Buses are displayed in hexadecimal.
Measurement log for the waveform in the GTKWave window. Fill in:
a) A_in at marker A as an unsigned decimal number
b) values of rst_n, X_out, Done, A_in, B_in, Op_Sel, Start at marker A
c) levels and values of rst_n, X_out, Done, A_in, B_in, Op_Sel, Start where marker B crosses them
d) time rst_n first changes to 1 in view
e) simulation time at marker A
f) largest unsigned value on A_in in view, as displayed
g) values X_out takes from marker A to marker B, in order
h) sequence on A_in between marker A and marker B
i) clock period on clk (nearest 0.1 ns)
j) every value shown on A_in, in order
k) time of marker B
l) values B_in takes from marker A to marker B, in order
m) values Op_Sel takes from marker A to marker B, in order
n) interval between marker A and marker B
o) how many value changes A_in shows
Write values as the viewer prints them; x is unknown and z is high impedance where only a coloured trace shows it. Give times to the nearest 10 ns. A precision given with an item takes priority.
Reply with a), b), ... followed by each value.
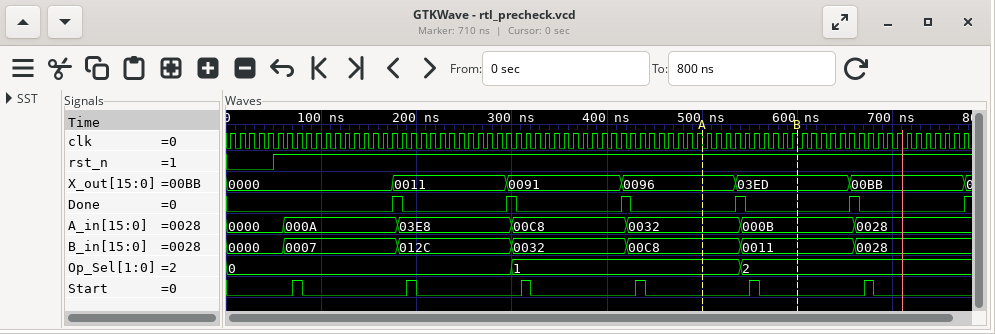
a) 50
b) rst_n=1, X_out=0096, Done=0, A_in=0032, B_in=00C8, Op_Sel=1, Start=0
c) rst_n=1, X_out=03ED, Done=0, A_in=000B, B_in=0011, Op_Sel=2, Start=0
d) 50 ns
e) 500 ns
f) 03E8
g) 0096, 03ED
h) 0032, 000B
i) 10 ns
j) 0000, 000A, 03E8, 00C8, 0032, 000B, 0028
k) 600 ns
l) 00C8, 0011
m) 1, 2
n) 100 ns
o) 6
